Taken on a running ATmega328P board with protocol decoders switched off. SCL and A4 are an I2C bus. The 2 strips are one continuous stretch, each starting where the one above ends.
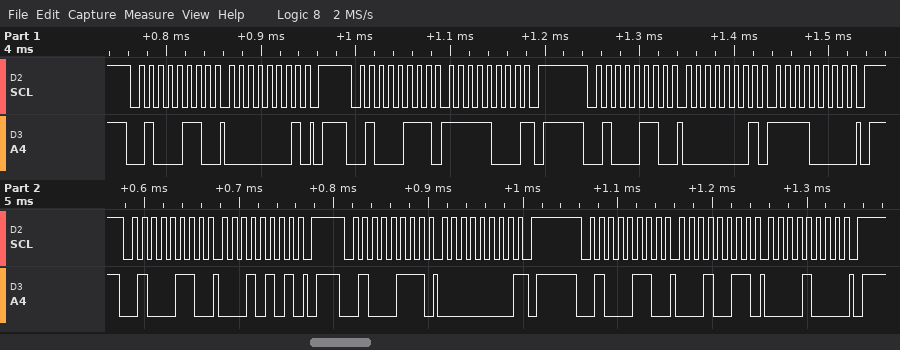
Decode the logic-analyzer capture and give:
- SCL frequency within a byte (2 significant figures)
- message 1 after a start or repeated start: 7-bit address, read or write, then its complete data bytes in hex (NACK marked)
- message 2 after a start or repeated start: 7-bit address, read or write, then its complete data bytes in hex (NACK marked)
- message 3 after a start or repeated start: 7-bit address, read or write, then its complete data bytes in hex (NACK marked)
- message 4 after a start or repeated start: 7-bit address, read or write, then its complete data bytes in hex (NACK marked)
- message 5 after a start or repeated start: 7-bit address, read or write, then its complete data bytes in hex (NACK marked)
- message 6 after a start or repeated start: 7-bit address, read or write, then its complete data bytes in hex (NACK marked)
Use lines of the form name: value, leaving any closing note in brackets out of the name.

SCL frequency within a byte: 100 kHz
message 1 after a start or repeated start: 7-bit address, read or write, then its complete data bytes in hex: 0x23 write: 01
message 2 after a start or repeated start: 7-bit address, read or write, then its complete data bytes in hex: 0x23 read: F8 NACK
message 3 after a start or repeated start: 7-bit address, read or write, then its complete data bytes in hex: 0x23 write: 01 F0
message 4 after a start or repeated start: 7-bit address, read or write, then its complete data bytes in hex: 0x23 write: 15
message 5 after a start or repeated start: 7-bit address, read or write, then its complete data bytes in hex: 0x23 read: 00 NACK
message 6 after a start or repeated start: 7-bit address, read or write, then its complete data bytes in hex: 0x23 write: 13 08
